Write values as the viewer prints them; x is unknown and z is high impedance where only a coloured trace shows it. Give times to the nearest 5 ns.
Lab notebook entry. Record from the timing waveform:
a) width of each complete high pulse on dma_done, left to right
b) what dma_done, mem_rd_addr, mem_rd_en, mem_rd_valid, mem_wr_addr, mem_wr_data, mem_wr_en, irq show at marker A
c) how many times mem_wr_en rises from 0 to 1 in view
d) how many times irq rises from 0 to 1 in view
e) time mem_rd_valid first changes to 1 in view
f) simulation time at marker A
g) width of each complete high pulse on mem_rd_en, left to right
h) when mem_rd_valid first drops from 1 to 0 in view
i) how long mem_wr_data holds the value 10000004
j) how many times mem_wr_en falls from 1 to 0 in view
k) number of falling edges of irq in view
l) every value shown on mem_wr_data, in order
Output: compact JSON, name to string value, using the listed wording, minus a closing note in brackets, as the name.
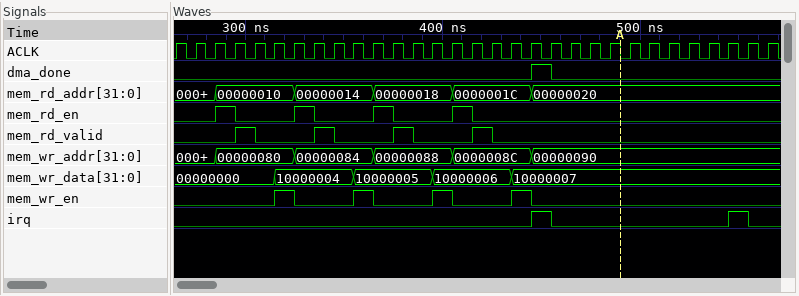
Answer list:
{"width of each complete high pulse on dma_done, left to right": "10 ns", "what dma_done, mem_rd_addr, mem_rd_en, mem_rd_valid, mem_wr_addr, mem_wr_data, mem_wr_en, irq show at marker A": "dma_done=0, mem_rd_addr=00000020, mem_rd_en=0, mem_rd_valid=0, mem_wr_addr=00000090, mem_wr_data=10000007, mem_wr_en=0, irq=0", "how many times mem_wr_en rises from 0 to 1 in view": "4", "how many times irq rises from 0 to 1 in view": "2", "time mem_rd_valid first changes to 1 in view": "295 ns", "simulation time at marker A": "490 ns", "width of each complete high pulse on mem_rd_en, left to right": "10 ns, 10 ns, 10 ns, 10 ns", "when mem_rd_valid first drops from 1 to 0 in view": "305 ns", "how long mem_wr_data holds the value 10000004": "40 ns", "how many times mem_wr_en falls from 1 to 0 in view": "4", "number of falling edges of irq in view": "2", "every value shown on mem_wr_data, in order": "00000000, 10000004, 10000005, 10000006, 10000007"}
